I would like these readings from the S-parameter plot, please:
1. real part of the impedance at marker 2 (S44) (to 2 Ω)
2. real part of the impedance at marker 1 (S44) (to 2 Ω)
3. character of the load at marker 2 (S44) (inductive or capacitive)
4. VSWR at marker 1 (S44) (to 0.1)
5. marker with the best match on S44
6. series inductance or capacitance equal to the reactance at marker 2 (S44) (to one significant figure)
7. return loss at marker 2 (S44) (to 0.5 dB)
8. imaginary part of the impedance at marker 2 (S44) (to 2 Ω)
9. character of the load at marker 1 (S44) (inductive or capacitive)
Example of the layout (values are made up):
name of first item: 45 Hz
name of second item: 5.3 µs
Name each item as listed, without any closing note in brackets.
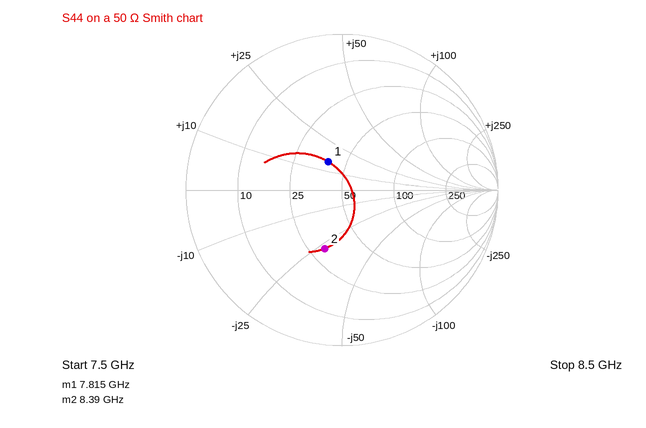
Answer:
real part of the impedance at marker 2 (S44): 30 Ω
real part of the impedance at marker 1 (S44): 40 Ω
character of the load at marker 2 (S44): capacitive
VSWR at marker 1 (S44): 1.5
marker with the best match on S44: marker 1
series inductance or capacitance equal to the reactance at marker 2 (S44): 700 fF
return loss at marker 2 (S44): 8.0 dB
imaginary part of the impedance at marker 2 (S44): -28 Ω
character of the load at marker 1 (S44): inductive
